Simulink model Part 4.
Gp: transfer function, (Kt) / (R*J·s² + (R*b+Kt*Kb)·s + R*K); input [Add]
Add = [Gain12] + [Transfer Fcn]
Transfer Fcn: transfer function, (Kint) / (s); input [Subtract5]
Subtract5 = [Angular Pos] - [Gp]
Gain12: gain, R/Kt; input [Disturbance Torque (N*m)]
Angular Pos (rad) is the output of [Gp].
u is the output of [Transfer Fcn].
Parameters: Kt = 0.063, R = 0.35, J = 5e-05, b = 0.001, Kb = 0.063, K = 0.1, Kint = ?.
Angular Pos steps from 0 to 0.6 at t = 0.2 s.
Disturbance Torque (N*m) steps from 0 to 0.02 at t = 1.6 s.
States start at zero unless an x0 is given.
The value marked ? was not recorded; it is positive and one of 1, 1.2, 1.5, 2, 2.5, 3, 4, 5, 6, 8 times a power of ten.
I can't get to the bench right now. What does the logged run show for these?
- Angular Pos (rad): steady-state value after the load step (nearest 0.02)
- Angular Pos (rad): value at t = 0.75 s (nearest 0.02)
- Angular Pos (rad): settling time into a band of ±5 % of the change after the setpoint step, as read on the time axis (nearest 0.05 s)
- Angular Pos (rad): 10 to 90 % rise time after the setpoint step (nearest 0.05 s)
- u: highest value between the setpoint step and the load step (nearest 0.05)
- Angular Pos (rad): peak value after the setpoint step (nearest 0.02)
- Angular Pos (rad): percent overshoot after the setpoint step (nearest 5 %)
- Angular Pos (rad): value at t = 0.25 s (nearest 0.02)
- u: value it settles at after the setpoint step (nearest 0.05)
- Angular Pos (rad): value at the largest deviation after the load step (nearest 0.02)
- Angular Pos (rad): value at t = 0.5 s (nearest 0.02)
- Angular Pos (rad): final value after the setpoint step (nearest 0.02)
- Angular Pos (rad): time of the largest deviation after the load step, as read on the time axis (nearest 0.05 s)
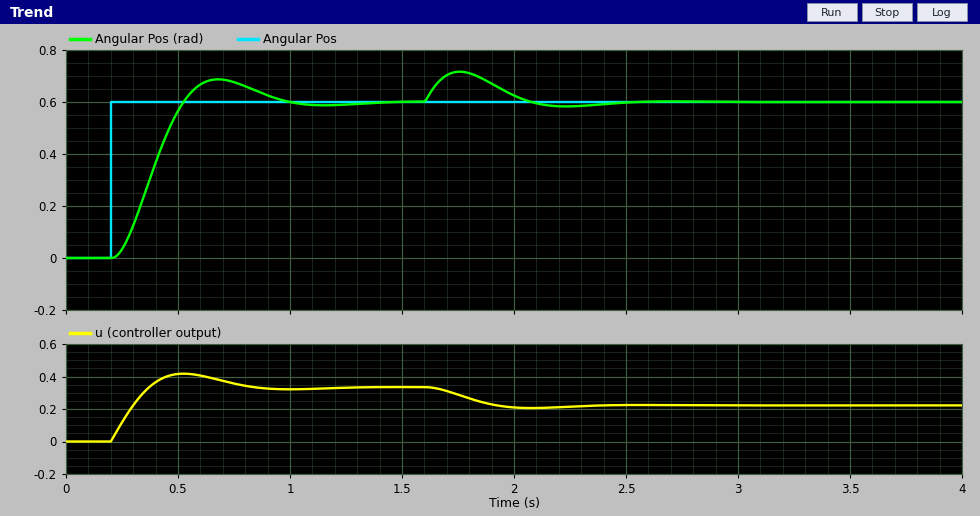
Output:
0.60
0.68
0.90 s
0.20 s
0.40
0.68
15 %
0.04
0.35
0.72
0.56
0.60
1.75 s
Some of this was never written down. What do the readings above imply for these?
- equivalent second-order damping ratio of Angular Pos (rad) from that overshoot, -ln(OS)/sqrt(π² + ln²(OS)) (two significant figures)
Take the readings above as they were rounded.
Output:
0.52
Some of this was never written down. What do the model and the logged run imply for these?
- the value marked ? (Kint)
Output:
4
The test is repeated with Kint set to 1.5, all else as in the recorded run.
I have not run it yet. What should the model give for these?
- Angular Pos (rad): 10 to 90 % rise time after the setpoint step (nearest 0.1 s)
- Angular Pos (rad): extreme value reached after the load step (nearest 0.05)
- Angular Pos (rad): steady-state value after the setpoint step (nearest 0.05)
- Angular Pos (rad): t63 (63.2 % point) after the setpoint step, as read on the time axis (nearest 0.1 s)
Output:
0.6 s
0.75
0.60
0.6 s
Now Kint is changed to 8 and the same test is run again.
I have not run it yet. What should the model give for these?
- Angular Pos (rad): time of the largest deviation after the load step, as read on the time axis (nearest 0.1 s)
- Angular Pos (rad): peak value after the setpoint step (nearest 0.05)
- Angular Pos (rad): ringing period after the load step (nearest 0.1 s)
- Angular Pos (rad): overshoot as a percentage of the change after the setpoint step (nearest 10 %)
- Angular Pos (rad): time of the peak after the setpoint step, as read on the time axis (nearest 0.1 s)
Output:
1.7 s
0.80
0.6 s
30 %
0.5 s
